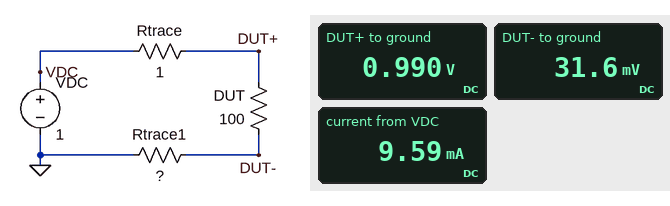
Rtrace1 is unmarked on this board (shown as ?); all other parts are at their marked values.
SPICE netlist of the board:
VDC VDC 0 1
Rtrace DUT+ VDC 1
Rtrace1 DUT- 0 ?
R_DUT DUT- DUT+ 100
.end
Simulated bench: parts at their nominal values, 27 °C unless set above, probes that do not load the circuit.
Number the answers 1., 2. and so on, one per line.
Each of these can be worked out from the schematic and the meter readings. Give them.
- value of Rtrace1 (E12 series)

1. 3.3 Ω
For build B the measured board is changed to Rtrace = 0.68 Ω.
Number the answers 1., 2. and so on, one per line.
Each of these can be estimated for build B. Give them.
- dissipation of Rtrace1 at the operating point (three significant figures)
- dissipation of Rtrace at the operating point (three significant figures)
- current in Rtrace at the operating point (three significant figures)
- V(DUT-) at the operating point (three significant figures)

1. 305 µW
2. 62.9 µW
3. 9.62 mA
4. 31.7 mV
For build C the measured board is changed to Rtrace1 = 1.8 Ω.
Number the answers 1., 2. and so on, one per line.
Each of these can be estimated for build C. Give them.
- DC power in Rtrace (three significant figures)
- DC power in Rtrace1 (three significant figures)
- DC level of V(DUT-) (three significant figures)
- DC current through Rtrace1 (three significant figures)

1. 94.6 µW
2. 170 µW
3. 17.5 mV
4. 9.73 mA
